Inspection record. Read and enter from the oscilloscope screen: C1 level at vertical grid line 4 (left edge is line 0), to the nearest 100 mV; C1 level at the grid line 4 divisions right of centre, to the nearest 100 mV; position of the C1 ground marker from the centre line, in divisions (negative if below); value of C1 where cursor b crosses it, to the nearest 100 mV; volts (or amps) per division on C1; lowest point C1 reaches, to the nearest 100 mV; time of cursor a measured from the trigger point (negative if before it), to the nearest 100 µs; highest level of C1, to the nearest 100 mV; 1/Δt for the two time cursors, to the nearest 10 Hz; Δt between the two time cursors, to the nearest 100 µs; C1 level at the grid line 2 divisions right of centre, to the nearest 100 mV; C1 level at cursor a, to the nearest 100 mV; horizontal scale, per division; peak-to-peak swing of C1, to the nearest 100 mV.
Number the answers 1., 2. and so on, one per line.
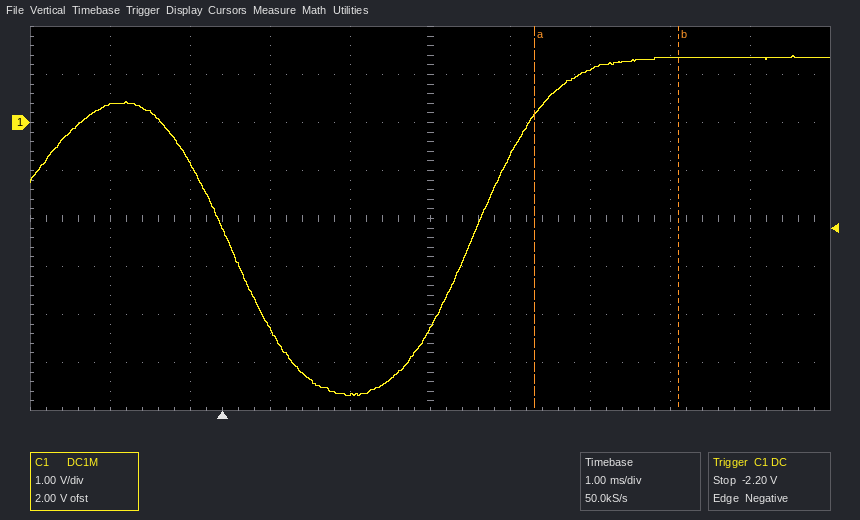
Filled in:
1. -5.7 V
2. 1.4 V
3. +2.0 div
4. 1.4 V
5. 1 V
6. -5.7 V
7. +3.9 ms
8. 1.4 V
9. 560 Hz
10. 1.8 ms
11. 1.1 V
12. 200 mV
13. 1 ms
14. 7.1 V
